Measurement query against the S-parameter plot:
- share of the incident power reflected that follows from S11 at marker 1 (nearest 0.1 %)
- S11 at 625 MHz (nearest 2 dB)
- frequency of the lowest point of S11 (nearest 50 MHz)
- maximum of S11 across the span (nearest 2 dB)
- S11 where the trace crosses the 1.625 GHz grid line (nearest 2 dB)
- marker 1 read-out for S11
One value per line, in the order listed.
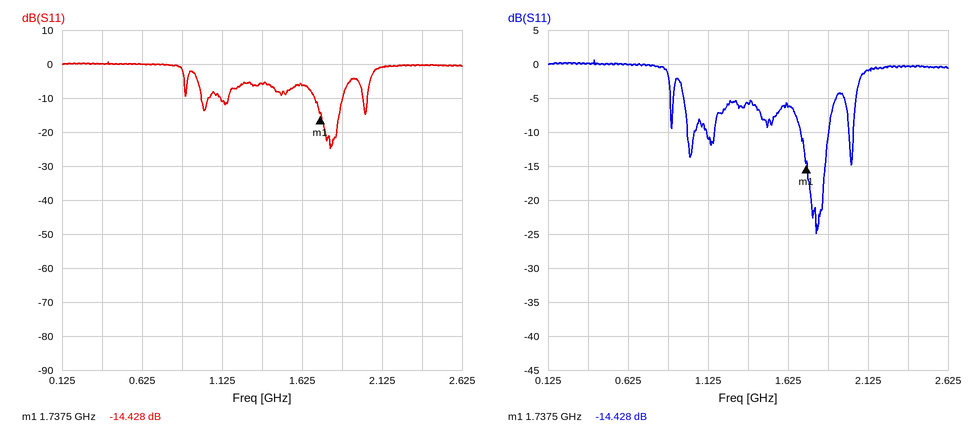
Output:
3.6 %
0 dB
1.80 GHz
0 dB
-6 dB
-14.428 dB
